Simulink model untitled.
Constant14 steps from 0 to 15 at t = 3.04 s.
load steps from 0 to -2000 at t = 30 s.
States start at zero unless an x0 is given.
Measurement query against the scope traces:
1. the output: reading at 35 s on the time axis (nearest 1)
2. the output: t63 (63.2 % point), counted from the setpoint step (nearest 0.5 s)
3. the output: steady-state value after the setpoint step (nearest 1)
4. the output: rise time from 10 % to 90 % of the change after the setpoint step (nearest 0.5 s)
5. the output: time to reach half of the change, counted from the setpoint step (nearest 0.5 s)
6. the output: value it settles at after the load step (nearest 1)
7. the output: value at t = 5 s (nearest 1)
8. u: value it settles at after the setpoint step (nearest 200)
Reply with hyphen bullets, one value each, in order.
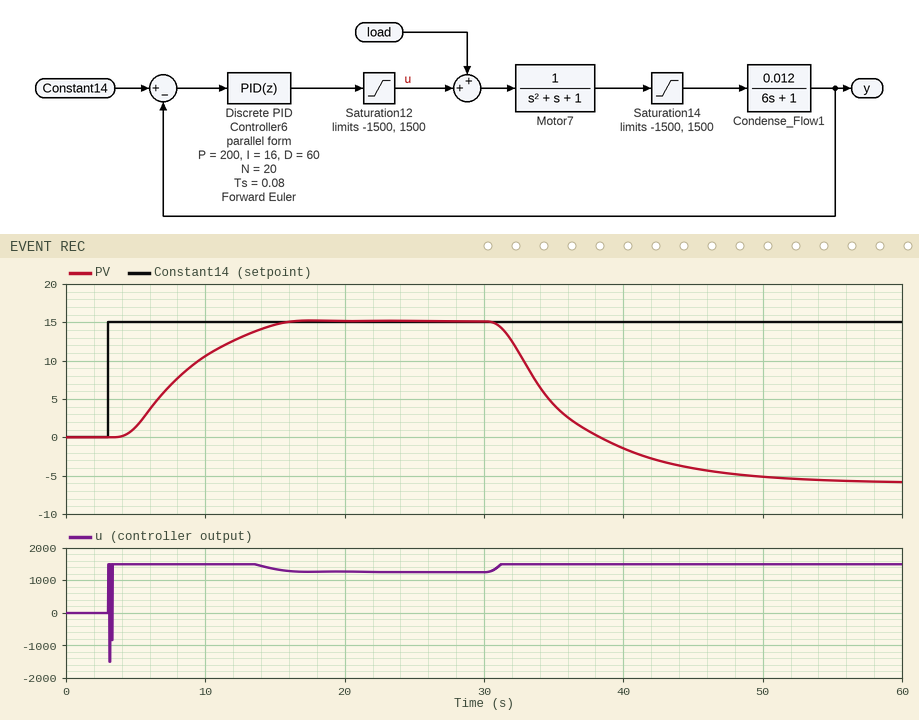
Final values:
- 4
- 6.0 s
- 15
- 8.0 s
- 5.0 s
- -6
- 1
- 1200
